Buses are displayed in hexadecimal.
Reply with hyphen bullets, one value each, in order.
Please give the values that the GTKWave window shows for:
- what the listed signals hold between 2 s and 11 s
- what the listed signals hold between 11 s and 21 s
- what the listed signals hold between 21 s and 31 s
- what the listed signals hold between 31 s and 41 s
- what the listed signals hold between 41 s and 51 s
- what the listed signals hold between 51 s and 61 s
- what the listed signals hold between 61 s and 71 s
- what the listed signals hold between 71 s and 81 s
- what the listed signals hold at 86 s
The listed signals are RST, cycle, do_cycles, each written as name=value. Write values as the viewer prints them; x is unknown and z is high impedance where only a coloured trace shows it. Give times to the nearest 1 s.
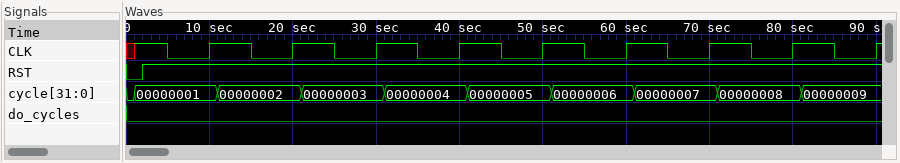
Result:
- RST=1, cycle=00000001, do_cycles=0
- RST=1, cycle=00000002, do_cycles=0
- RST=1, cycle=00000003, do_cycles=0
- RST=1, cycle=00000004, do_cycles=0
- RST=1, cycle=00000005, do_cycles=0
- RST=1, cycle=00000006, do_cycles=0
- RST=1, cycle=00000007, do_cycles=0
- RST=1, cycle=00000008, do_cycles=0
- RST=1, cycle=00000009, do_cycles=0
